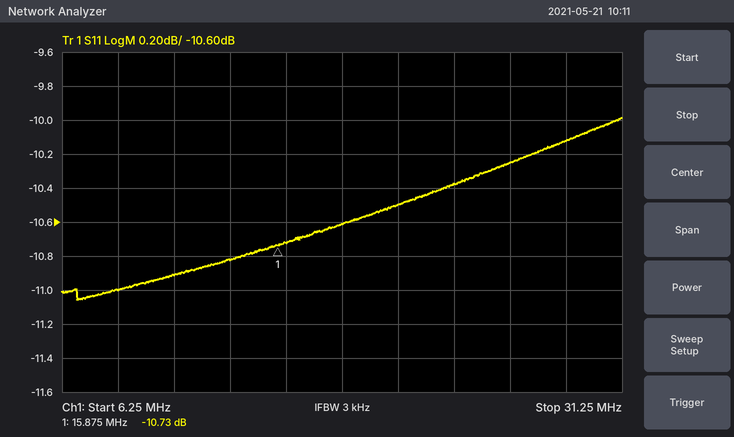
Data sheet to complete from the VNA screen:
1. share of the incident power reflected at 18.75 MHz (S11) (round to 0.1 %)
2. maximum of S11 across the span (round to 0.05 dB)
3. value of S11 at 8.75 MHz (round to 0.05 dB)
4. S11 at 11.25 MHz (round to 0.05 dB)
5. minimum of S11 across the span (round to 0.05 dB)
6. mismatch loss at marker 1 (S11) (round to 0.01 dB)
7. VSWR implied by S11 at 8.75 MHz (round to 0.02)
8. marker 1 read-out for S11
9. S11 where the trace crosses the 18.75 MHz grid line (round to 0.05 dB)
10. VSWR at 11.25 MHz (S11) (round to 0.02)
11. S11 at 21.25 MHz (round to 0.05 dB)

8.7 %
-10.00 dB
-11.00 dB
-10.90 dB
-11.05 dB
0.38 dB
1.78
-10.73 dB
-10.60 dB
1.80
-10.50 dB
